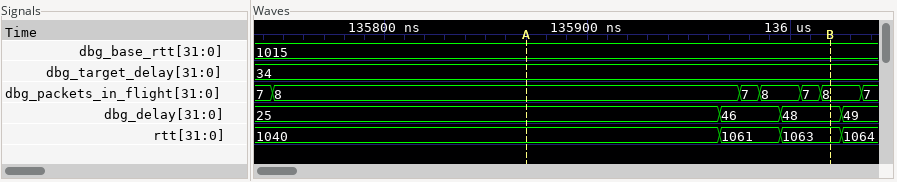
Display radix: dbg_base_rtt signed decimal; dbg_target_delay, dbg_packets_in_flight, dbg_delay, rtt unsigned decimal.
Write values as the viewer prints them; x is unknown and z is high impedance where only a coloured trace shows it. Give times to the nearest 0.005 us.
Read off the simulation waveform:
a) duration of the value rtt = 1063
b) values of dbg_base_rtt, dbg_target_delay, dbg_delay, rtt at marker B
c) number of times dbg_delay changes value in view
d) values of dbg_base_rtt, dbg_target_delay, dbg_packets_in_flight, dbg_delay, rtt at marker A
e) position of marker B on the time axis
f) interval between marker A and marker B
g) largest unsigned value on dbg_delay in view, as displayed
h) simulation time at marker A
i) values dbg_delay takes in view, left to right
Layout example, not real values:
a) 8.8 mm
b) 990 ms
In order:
a) 0.03 us
b) dbg_base_rtt=1015, dbg_target_delay=34, dbg_delay=48, rtt=1063
c) 3
d) dbg_base_rtt=1015, dbg_target_delay=34, dbg_packets_in_flight=8, dbg_delay=25, rtt=1040
e) 136.02 us
f) 0.15 us
g) 49
h) 135.87 us
i) 25, 46, 48, 49
